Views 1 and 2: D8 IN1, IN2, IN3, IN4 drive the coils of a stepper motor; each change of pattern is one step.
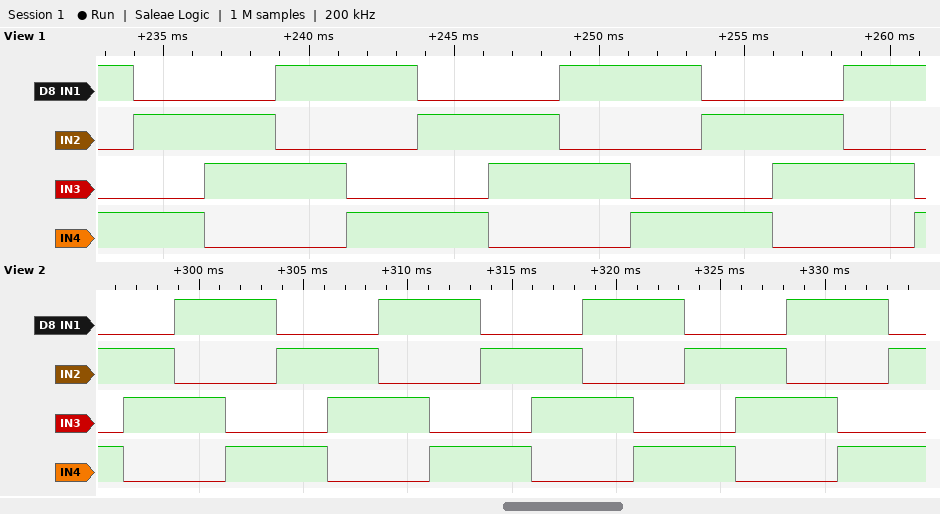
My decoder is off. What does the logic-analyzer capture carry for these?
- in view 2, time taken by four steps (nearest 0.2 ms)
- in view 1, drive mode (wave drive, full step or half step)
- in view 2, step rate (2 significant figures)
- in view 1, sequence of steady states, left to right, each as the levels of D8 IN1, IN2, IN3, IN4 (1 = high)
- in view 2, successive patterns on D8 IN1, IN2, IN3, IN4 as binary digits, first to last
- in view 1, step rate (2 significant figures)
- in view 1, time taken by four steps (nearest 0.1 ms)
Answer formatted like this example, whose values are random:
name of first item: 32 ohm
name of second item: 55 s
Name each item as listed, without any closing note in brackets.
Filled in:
in view 2, time taken by four steps: 9.8 ms
in view 1, drive mode: full step
in view 2, step rate: 410 steps/s
in view 1, sequence of steady states, left to right, each as the levels of D8 IN1, IN2, IN3, IN4: 1001 0101 0110 1010 1001 0101 0110 1010 1001 0101 0110 1010 1001
in view 2, successive patterns on D8 IN1, IN2, IN3, IN4 as binary digits, first to last: 0101 0110 1010 1001 0101 0110 1010 1001 0101 0110 1010 1001 0101 0110 1010 1001 0101
in view 1, step rate: 410 steps/s
in view 1, time taken by four steps: 9.8 ms
